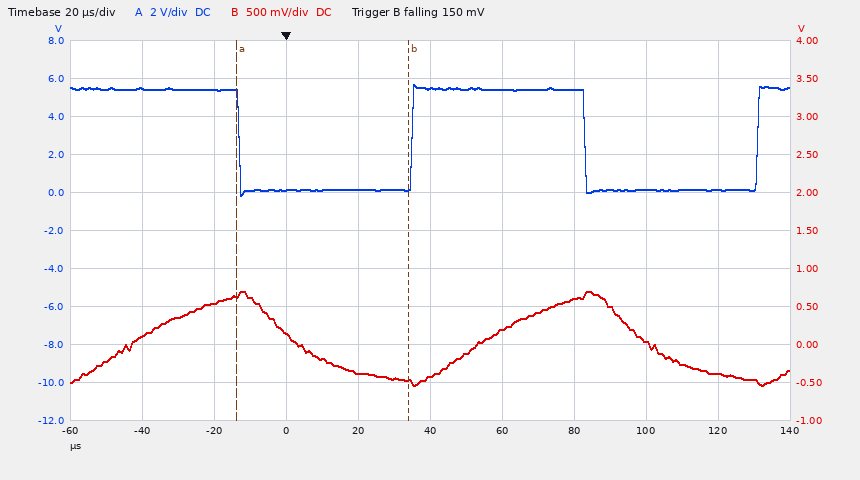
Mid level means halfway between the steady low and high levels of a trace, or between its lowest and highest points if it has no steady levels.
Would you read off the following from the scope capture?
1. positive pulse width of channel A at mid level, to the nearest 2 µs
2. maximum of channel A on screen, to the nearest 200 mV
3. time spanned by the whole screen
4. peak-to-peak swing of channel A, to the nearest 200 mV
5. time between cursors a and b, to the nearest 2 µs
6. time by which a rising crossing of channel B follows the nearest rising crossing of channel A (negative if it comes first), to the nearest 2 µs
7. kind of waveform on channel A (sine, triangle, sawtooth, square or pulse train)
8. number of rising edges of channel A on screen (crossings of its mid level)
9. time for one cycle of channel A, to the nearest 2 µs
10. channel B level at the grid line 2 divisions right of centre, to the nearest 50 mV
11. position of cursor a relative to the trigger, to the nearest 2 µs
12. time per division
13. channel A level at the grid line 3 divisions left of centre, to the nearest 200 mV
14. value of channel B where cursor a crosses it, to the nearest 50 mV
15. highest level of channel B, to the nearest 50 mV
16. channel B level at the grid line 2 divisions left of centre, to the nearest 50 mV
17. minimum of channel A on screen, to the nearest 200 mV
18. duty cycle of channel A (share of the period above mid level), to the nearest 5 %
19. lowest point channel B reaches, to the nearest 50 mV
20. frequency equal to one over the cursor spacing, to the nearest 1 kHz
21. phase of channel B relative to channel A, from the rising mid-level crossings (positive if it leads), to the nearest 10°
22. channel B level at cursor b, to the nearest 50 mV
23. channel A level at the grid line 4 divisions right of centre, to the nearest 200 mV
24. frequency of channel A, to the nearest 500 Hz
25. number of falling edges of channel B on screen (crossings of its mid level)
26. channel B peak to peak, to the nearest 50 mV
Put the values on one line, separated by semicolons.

48 µs; 5.6 V; 200 µs; 5.8 V; 48 µs; +20 µs; square; 2; 96 µs; 600 mV; -14 µs; 20 µs; 5.4 V; 650 mV; 700 mV; 150 mV; -200 mV; 50 %; -550 mV; 21 kHz; -80°; -500 mV; 200 mV; 10.5 kHz; 2; 1.25 V
